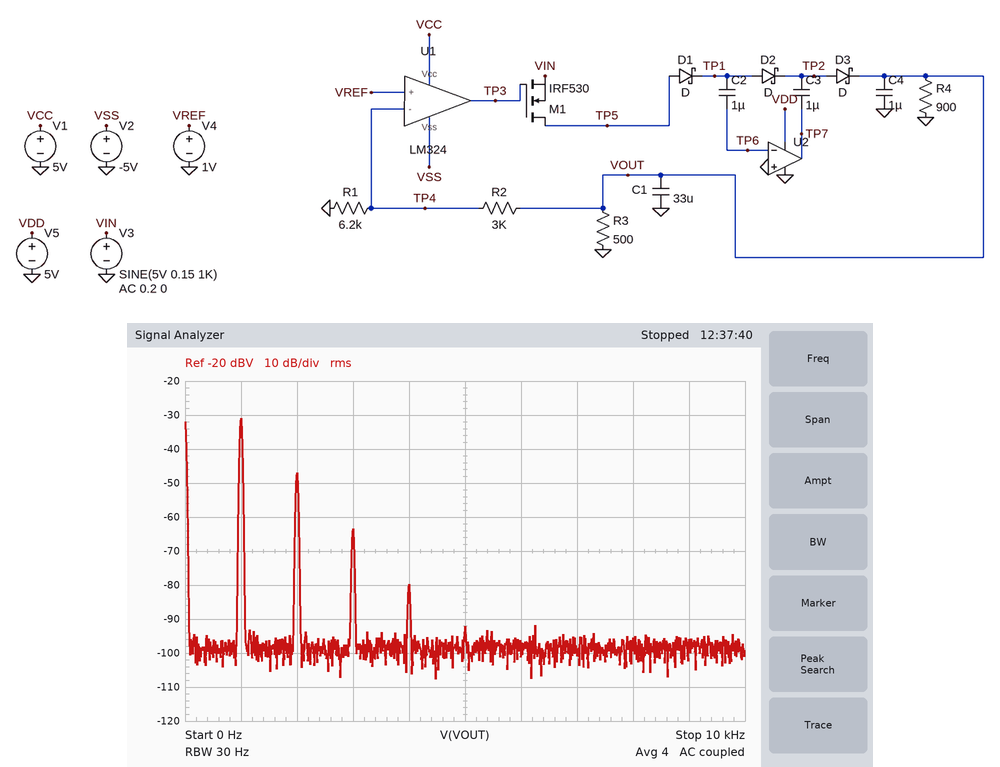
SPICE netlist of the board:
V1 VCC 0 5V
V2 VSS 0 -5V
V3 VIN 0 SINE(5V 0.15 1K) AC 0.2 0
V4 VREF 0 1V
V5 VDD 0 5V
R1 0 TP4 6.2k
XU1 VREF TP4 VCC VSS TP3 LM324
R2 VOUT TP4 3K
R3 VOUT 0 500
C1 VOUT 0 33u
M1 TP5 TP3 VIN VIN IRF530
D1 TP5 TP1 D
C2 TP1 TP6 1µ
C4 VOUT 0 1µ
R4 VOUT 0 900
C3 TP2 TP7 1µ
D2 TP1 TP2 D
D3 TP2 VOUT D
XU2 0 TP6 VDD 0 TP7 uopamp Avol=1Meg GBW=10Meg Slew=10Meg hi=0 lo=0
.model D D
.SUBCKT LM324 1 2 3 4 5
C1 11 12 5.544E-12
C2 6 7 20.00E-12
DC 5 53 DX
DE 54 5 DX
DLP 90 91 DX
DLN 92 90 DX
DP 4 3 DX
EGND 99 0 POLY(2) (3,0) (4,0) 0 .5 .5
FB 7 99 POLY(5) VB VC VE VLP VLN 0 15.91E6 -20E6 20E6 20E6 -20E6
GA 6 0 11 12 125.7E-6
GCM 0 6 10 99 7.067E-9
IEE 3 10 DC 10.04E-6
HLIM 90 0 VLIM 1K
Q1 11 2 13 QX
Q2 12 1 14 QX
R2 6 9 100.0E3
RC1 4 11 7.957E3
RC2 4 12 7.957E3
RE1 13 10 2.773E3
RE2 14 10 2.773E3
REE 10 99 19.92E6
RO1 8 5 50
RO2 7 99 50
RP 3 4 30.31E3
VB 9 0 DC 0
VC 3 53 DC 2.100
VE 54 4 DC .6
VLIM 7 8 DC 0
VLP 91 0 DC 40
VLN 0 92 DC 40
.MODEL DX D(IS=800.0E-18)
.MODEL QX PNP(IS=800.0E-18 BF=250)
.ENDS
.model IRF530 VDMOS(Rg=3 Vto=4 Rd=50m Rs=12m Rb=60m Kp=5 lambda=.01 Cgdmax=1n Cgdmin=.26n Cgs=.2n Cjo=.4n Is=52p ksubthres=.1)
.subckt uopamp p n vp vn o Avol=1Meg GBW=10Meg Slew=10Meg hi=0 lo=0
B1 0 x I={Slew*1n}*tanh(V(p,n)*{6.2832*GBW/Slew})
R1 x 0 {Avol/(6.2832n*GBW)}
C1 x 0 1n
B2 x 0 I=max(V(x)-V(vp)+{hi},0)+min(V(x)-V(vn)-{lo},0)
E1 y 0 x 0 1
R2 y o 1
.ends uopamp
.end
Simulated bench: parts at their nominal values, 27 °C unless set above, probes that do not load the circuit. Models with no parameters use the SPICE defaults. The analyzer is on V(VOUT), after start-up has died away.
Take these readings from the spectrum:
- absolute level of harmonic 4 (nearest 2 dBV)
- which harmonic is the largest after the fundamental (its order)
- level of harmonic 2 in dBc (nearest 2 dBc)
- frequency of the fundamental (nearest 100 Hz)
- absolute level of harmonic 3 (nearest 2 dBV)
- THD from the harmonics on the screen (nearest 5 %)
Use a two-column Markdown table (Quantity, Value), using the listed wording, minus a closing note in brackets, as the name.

| Quantity | Value |
|---|---|
| absolute level of harmonic 4 | -80 dBV |
| which harmonic is the largest after the fundamental | 2 |
| level of harmonic 2 in dBc | -16 dBc |
| frequency of the fundamental | 1.0 kHz |
| absolute level of harmonic 3 | -64 dBV |
| THD from the harmonics on the screen | 15 % |
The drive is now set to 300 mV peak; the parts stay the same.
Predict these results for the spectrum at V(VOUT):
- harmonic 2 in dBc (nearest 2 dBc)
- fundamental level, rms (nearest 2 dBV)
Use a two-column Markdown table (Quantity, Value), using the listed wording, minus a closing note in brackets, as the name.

| Quantity | Value |
|---|---|
| harmonic 2 in dBc | -12 dBc |
| fundamental level, rms | -28 dBV |
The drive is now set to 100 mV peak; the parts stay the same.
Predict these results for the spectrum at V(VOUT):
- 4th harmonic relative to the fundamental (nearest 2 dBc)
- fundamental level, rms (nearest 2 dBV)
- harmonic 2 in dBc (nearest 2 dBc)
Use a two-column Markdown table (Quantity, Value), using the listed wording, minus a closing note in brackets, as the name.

| Quantity | Value |
|---|---|
| 4th harmonic relative to the fundamental | -58 dBc |
| fundamental level, rms | -34 dBV |
| harmonic 2 in dBc | -20 dBc |
